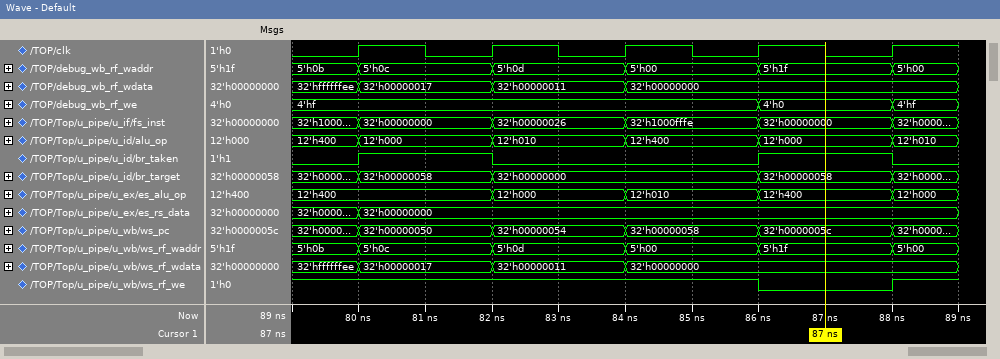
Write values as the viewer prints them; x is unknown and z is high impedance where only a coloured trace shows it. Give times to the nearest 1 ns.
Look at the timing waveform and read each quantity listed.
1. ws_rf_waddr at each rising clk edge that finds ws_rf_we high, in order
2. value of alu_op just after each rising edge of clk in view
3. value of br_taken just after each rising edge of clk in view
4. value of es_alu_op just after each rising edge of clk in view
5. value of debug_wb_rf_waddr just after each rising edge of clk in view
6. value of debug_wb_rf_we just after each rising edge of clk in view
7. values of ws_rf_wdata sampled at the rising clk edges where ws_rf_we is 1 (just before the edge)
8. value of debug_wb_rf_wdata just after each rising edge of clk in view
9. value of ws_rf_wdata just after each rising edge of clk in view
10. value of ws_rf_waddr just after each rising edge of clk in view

5'h0b, 5'h0c, 5'h0d, 5'h00
12'h000, 12'h010, 12'h400, 12'h000, 12'h010
1 0 0 1 0
12'h400, 12'h000, 12'h010, 12'h400, 12'h000
5'h0c, 5'h0d, 5'h00, 5'h1f, 5'h00
4'hf, 4'hf, 4'hf, 4'h0, 4'hf
32'hffffffee, 32'h00000017, 32'h00000011, 32'h00000000
32'h00000017, 32'h00000011, 32'h00000000, 32'h00000000, 32'h00000000
32'h00000017, 32'h00000011, 32'h00000000, 32'h00000000, 32'h00000000
5'h0c, 5'h0d, 5'h00, 5'h1f, 5'h00
